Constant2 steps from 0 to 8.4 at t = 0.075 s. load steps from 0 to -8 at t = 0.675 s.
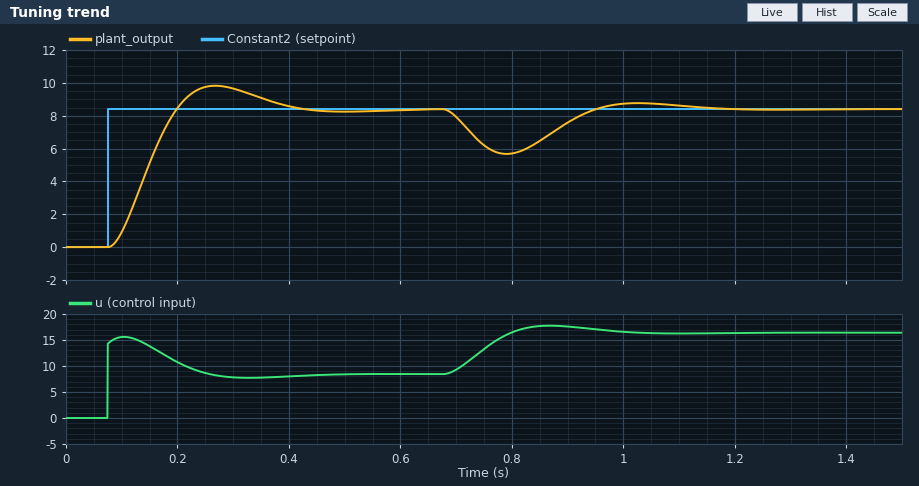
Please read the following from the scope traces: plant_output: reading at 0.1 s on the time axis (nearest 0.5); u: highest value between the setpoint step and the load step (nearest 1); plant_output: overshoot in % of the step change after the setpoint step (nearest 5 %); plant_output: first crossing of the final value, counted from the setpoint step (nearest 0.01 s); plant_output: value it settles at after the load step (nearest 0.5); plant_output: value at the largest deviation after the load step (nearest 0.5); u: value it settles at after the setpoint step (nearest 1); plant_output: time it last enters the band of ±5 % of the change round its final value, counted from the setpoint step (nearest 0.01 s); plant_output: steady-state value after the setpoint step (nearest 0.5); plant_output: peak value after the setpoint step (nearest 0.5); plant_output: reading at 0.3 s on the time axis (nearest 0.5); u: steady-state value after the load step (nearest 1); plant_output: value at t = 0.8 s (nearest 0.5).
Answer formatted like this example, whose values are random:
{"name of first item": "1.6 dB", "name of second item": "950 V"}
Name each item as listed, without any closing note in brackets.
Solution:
{"plant_output: reading at 0.1 s on the time axis": "1.0", "u: highest value between the setpoint step and the load step": "16", "plant_output: overshoot in % of the step change after the setpoint step": "15 %", "plant_output: first crossing of the final value, counted from the setpoint step": "0.12 s", "plant_output: value it settles at after the load step": "8.5", "plant_output: value at the largest deviation after the load step": "5.5", "u: value it settles at after the setpoint step": "8", "plant_output: time it last enters the band of ±5 % of the change round its final value, counted from the setpoint step": "0.30 s", "plant_output: steady-state value after the setpoint step": "8.5", "plant_output: peak value after the setpoint step": "10.0", "plant_output: reading at 0.3 s on the time axis": "9.5", "u: steady-state value after the load step": "16", "plant_output: value at t = 0.8 s": "5.5"}
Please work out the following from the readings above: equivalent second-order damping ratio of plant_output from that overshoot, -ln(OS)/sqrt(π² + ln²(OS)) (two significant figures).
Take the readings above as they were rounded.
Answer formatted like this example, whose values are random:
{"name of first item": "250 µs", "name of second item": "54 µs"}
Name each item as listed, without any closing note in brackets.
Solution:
{"equivalent second-order damping ratio of plant_output from that overshoot, -ln(OS)/sqrt(π² + ln²(OS))": "0.52"}
